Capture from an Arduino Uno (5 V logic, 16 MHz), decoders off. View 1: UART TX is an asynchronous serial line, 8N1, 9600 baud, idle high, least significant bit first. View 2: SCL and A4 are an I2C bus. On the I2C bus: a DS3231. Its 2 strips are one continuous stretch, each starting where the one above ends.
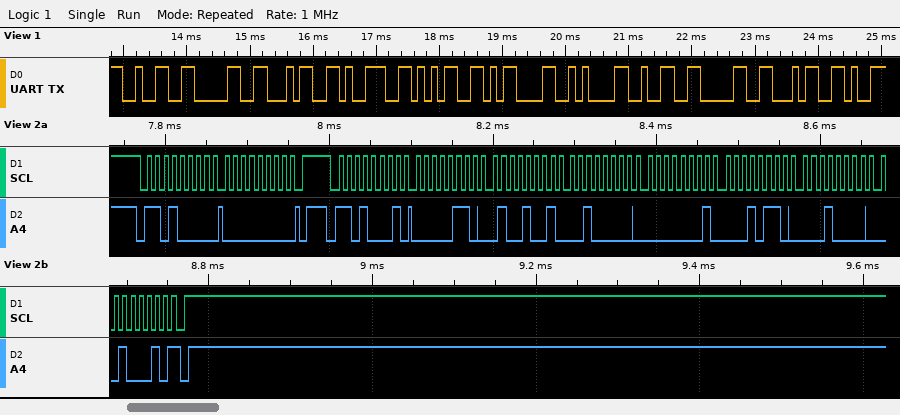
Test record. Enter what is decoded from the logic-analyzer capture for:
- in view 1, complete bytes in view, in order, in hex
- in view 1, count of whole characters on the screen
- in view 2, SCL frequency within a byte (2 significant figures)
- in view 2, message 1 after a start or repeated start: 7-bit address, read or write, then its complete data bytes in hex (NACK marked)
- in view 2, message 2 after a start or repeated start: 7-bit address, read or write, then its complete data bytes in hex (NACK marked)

32 30 34 39 35 0D 0A 32 30 34
10
100 kHz
0x68 write: 00
0x68 read: 06 49 20 01 16 10 22 NACK
